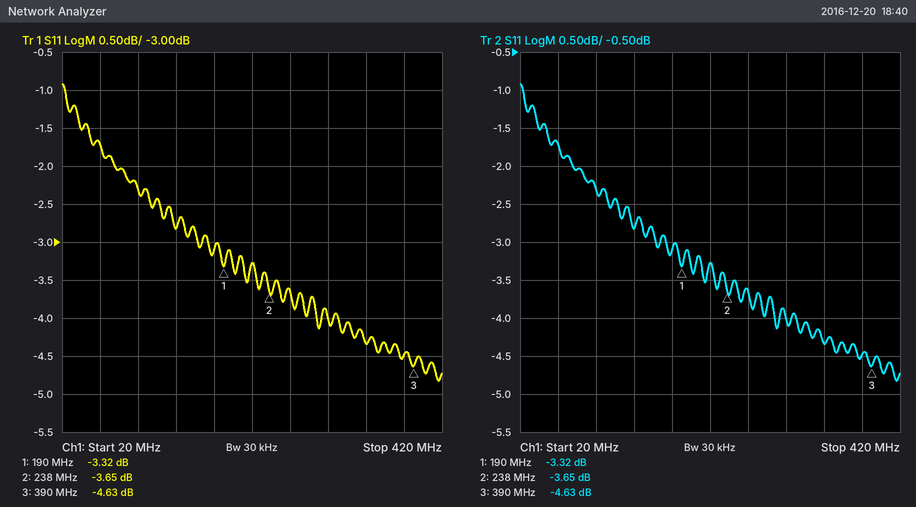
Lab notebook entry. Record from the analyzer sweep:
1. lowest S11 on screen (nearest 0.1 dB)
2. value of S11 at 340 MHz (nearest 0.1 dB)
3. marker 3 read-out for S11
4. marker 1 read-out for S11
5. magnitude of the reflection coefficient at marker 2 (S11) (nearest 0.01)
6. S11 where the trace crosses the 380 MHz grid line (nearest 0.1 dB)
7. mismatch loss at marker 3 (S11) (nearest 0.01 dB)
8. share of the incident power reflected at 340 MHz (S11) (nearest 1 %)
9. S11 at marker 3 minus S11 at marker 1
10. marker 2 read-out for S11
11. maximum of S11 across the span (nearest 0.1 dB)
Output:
-4.8 dB
-4.3 dB
-4.63 dB
-3.32 dB
0.66
-4.5 dB
1.83 dB
37 %
-1.31 dB
-3.65 dB
-0.9 dB
